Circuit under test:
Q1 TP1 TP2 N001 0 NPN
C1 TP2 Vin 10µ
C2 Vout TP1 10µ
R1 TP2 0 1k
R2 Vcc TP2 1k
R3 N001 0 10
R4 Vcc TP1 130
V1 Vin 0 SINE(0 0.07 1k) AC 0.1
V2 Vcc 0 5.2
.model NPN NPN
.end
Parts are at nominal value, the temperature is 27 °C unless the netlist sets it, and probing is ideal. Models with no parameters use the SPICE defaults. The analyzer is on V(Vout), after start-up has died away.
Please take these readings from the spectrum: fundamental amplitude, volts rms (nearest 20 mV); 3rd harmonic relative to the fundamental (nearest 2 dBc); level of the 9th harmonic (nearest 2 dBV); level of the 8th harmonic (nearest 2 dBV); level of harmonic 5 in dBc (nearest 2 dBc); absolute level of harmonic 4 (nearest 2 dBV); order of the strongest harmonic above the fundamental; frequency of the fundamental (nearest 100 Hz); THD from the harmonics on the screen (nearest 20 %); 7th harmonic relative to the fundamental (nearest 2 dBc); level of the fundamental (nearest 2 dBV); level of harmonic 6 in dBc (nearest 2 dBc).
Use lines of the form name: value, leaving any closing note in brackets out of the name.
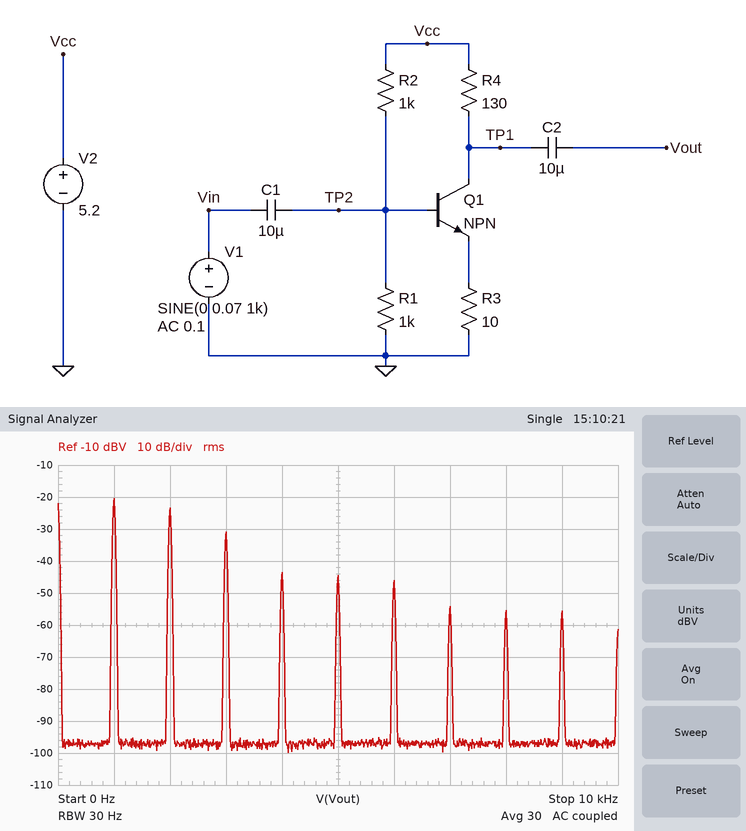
fundamental amplitude, volts rms: 100 mV
3rd harmonic relative to the fundamental: -10 dBc
level of the 9th harmonic: -56 dBV
level of the 8th harmonic: -56 dBV
level of harmonic 5 in dBc: -24 dBc
absolute level of harmonic 4: -44 dBV
order of the strongest harmonic above the fundamental: 2
frequency of the fundamental: 1.0 kHz
THD from the harmonics on the screen: 80 %
7th harmonic relative to the fundamental: -34 dBc
level of the fundamental: -20 dBV
level of harmonic 6 in dBc: -26 dBc
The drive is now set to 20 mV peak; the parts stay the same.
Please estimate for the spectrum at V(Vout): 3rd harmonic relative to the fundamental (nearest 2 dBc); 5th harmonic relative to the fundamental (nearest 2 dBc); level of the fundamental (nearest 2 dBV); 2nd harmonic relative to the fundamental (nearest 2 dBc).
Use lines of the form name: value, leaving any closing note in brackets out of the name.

3rd harmonic relative to the fundamental: -8 dBc
5th harmonic relative to the fundamental: -42 dBc
level of the fundamental: -70 dBV
2nd harmonic relative to the fundamental: 8 dBc
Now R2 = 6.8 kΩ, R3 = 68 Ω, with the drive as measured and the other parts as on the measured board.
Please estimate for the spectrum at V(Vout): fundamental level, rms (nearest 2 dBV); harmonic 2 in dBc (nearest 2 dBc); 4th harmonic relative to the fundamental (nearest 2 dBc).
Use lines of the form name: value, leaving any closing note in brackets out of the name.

fundamental level, rms: -44 dBV
harmonic 2 in dBc: -6 dBc
4th harmonic relative to the fundamental: -32 dBc
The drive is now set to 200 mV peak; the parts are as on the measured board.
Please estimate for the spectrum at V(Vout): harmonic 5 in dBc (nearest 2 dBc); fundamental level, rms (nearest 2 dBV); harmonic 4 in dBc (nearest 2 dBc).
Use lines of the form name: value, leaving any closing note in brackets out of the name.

harmonic 5 in dBc: -28 dBc
fundamental level, rms: 0 dBV
harmonic 4 in dBc: -30 dBc
